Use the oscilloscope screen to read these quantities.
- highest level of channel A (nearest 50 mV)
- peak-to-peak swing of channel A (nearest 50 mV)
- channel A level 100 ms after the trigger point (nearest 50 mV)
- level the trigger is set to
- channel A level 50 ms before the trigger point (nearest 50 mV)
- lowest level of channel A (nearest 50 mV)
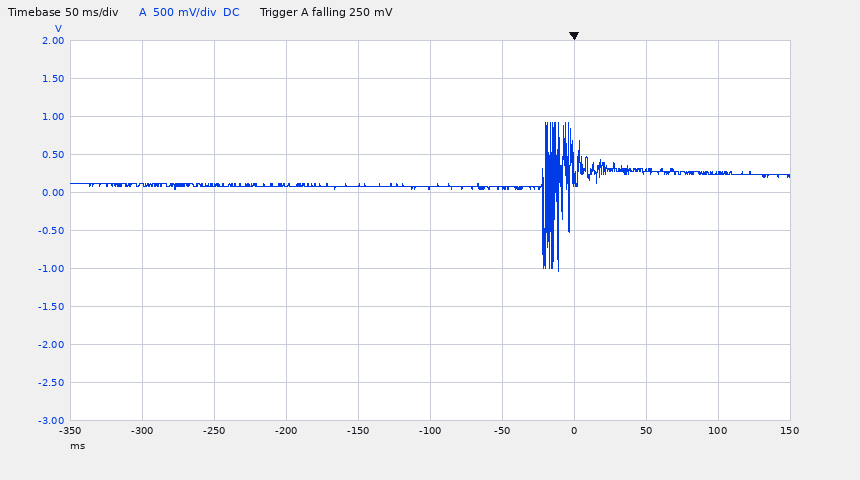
900 mV
1.95 V
250 mV
250 mV
50 mV
-1.05 V
